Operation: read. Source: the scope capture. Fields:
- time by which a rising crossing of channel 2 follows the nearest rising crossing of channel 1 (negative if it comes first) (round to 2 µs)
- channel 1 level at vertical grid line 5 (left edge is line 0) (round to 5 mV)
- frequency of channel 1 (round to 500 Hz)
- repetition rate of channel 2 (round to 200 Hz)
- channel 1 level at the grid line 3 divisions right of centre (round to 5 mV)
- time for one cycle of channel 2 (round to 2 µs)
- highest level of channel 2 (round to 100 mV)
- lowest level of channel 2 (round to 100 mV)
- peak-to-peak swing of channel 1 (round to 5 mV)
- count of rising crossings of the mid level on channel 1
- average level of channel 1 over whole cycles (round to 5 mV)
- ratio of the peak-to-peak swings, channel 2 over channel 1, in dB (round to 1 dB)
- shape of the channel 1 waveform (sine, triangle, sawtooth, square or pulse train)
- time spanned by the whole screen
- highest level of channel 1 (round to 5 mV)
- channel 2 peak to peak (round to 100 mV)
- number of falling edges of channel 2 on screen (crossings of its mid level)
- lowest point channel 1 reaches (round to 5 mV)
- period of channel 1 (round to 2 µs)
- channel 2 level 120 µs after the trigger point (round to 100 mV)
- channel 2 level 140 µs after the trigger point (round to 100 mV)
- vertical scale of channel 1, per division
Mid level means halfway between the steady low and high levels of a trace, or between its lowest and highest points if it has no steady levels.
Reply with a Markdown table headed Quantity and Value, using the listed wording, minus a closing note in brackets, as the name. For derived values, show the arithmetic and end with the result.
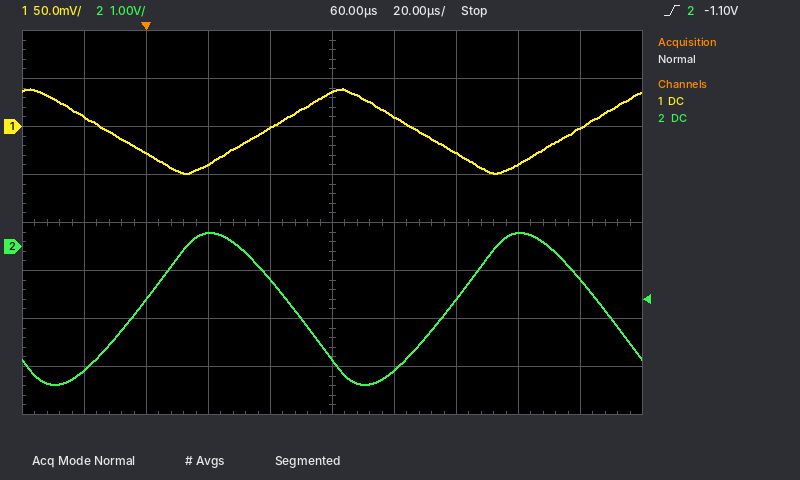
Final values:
| Quantity | Value |
|---|---|
| time by which a rising crossing of channel 2 follows the nearest rising crossing of channel 1 (negative if it comes first) | -40 µs |
| channel 1 level at vertical grid line 5 (left edge is line 0) | 35 mV |
| frequency of channel 1 | 1 / 100 µs ≈ 10.0 kHz |
| repetition rate of channel 2 | 1 / 100 µs ≈ 10.0 kHz |
| channel 1 level at the grid line 3 divisions right of centre | -40 mV |
| time for one cycle of channel 2 | 100 µs |
| highest level of channel 2 | 300 mV |
| lowest level of channel 2 | -2.9 V |
| peak-to-peak swing of channel 1 | 40 mV − (-50 mV) = 90 mV |
| count of rising crossings of the mid level on channel 1 | 2 |
| average level of channel 1 over whole cycles | (40 mV + (-50 mV)) / 2 ≈ -5 mV |
| ratio of the peak-to-peak swings, channel 2 over channel 1, in dB | 20 log10(3.2 V / 90 mV) ≈ 31 dB |
| shape of the channel 1 waveform | triangle |
| time spanned by the whole screen | 200 µs |
| highest level of channel 1 | 40 mV |
| channel 2 peak to peak | 300 mV − (-2.9 V) = 3.2 V |
| number of falling edges of channel 2 on screen | 2 |
| lowest point channel 1 reaches | -50 mV |
| period of channel 1 | 100 µs |
| channel 2 level 120 µs after the trigger point | 300 mV |
| channel 2 level 140 µs after the trigger point | -700 mV |
| vertical scale of channel 1, per division | 50 mV |
